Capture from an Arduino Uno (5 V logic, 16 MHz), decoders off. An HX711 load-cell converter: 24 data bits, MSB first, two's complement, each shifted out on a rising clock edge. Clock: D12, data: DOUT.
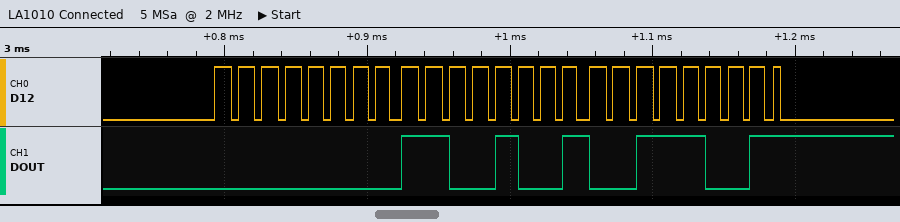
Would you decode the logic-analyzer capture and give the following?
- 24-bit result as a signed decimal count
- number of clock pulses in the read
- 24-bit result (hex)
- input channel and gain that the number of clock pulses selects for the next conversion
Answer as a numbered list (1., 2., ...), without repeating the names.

1. 51513
2. 25
3. 0x00C939
4. channel A, gain 128
